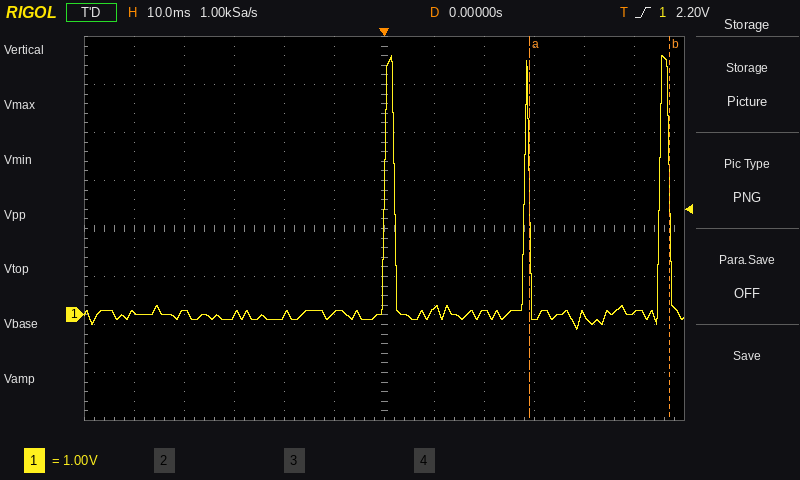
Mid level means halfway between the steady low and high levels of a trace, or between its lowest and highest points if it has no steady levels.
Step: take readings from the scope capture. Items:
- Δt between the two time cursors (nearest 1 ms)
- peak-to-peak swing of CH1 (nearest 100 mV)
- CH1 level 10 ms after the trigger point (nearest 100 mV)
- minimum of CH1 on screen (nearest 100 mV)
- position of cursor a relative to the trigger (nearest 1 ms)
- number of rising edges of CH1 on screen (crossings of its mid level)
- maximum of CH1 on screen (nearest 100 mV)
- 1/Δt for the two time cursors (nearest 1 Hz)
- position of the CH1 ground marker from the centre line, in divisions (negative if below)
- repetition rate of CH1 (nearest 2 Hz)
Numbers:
28 ms
5.7 V
100 mV
-300 mV
+29 ms
3
5.4 V
36 Hz
-1.8 div
36 Hz
